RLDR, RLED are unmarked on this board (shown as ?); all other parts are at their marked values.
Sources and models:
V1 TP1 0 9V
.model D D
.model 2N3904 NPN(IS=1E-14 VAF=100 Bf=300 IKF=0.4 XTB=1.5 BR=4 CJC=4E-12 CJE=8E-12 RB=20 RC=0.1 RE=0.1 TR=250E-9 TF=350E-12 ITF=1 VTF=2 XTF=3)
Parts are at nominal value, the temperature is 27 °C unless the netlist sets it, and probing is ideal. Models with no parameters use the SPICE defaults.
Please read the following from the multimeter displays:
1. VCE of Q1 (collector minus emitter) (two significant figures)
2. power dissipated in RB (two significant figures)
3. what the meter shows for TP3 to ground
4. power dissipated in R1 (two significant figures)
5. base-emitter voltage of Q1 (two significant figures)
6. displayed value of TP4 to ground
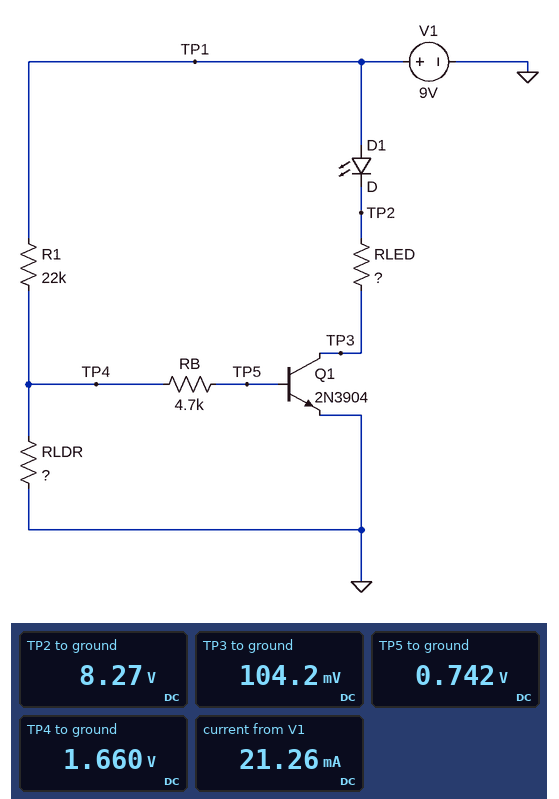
100 mV
180 µW
104.2 mV
2.4 mW
740 mV
1.660 V
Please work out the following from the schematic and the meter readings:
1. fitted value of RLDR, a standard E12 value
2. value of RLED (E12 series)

12 kΩ
390 Ω
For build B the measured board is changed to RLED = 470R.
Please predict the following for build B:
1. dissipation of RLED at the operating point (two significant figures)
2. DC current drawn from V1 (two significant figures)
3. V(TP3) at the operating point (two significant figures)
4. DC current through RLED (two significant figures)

140 mW
18 mA
96 mV
17 mA
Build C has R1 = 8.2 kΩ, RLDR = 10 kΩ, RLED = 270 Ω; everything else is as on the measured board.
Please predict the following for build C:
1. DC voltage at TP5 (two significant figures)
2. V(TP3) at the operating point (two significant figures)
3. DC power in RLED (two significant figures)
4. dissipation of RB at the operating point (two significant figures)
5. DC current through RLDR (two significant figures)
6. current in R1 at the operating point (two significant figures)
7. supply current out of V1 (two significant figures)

760 mV
90 mV
250 mW
970 µW
290 µA
740 µA
31 mA
